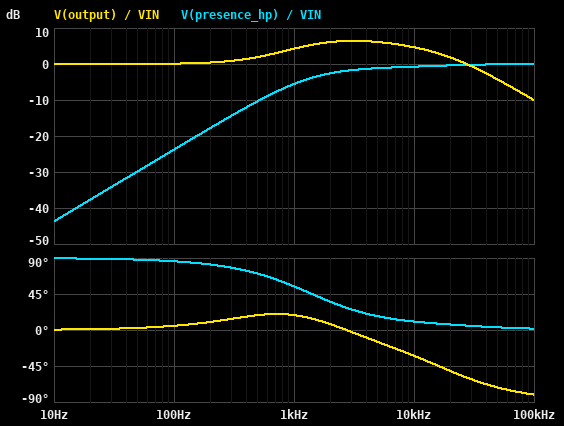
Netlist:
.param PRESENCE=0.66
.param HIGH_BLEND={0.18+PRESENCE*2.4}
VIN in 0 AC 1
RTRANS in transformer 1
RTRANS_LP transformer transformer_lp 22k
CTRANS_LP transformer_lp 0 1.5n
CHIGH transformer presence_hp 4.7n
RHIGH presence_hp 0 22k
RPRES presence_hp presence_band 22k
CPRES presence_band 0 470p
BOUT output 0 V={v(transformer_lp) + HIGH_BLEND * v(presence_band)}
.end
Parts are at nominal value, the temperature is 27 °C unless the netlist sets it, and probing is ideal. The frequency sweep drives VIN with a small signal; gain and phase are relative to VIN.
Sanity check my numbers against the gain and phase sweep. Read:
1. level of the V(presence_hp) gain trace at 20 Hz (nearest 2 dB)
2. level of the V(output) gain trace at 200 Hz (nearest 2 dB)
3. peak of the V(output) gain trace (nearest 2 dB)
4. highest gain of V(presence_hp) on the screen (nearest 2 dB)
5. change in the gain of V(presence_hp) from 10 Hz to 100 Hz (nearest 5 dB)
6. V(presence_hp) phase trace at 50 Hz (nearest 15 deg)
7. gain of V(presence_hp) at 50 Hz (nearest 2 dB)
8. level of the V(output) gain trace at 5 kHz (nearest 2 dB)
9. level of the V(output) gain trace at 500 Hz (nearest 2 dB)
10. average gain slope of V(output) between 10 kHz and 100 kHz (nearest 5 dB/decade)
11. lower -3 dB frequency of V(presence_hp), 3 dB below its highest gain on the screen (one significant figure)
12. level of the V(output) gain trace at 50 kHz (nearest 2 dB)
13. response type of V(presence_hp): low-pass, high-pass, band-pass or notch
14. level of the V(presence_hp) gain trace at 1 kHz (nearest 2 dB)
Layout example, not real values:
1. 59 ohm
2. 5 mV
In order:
1. -38 dB
2. 0 dB
3. 6 dB
4. 0 dB
5. 20 dB
6. 90 deg
7. -30 dB
8. 6 dB
9. 2 dB
10. -15 dB/decade
11. 2 kHz
12. -4 dB
13. high-pass
14. -6 dB
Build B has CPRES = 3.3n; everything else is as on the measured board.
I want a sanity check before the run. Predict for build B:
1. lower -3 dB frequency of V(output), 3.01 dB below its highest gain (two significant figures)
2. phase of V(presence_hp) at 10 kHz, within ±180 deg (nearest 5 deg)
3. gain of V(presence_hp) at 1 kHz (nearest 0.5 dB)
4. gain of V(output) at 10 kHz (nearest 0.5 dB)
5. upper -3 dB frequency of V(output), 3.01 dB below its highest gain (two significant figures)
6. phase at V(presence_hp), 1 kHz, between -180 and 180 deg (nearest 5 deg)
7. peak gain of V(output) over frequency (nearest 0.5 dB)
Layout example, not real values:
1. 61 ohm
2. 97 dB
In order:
1. 310 Hz
2. 15 deg
3. -7.5 dB
4. -2.0 dB
5. 5.8 kHz
6. 50 deg
7. 4.5 dB
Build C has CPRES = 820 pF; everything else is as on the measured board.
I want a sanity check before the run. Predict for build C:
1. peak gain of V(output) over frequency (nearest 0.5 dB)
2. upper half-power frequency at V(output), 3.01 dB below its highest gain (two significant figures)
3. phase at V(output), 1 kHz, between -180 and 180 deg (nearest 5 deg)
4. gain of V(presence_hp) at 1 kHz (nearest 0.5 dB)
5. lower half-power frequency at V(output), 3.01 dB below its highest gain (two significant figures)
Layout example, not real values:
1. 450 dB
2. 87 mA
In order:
1. 6.0 dB
2. 10 kHz
3. 15 deg
4. -6.0 dB
5. 710 Hz
